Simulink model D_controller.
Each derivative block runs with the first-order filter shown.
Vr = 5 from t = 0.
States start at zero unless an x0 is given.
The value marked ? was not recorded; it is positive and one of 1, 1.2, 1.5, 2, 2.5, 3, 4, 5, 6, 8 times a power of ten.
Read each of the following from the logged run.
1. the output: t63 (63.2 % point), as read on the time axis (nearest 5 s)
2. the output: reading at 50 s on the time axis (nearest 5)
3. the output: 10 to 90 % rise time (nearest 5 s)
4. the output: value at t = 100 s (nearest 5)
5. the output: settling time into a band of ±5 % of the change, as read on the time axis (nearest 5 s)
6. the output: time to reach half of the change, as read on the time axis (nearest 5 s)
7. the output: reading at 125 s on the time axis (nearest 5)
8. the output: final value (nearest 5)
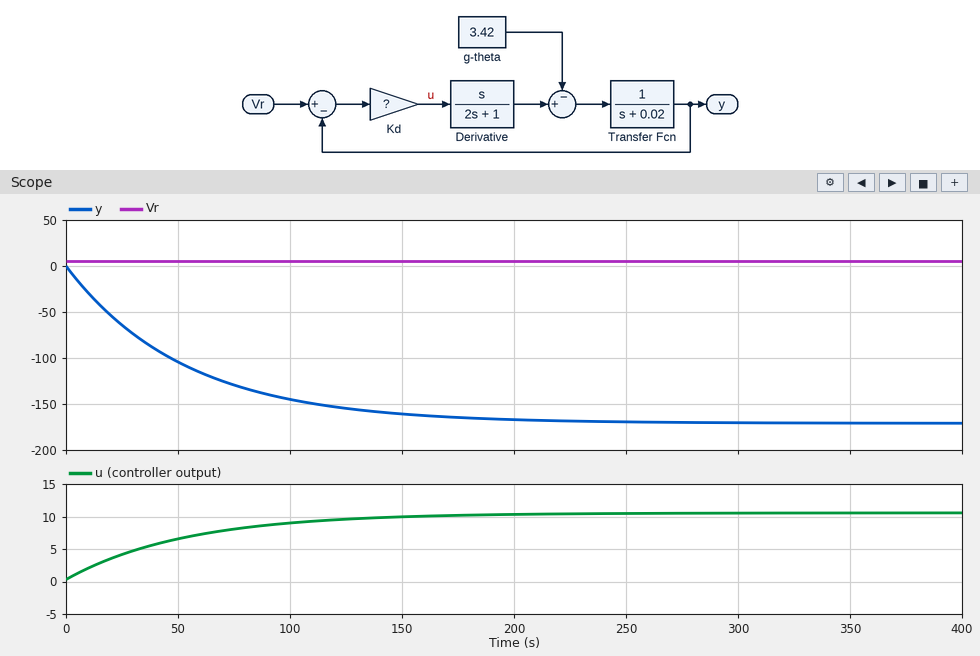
55 s
-105
115 s
-145
160 s
35 s
-155
-170
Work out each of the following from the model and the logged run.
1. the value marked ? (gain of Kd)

0.06
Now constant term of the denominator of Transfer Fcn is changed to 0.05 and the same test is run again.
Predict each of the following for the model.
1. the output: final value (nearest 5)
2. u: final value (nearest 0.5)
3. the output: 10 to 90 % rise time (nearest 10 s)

-70
4.5
50 s
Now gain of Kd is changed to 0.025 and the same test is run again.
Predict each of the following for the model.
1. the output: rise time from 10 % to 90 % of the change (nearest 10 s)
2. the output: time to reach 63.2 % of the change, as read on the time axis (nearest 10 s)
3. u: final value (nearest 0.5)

110 s
50 s
4.5
